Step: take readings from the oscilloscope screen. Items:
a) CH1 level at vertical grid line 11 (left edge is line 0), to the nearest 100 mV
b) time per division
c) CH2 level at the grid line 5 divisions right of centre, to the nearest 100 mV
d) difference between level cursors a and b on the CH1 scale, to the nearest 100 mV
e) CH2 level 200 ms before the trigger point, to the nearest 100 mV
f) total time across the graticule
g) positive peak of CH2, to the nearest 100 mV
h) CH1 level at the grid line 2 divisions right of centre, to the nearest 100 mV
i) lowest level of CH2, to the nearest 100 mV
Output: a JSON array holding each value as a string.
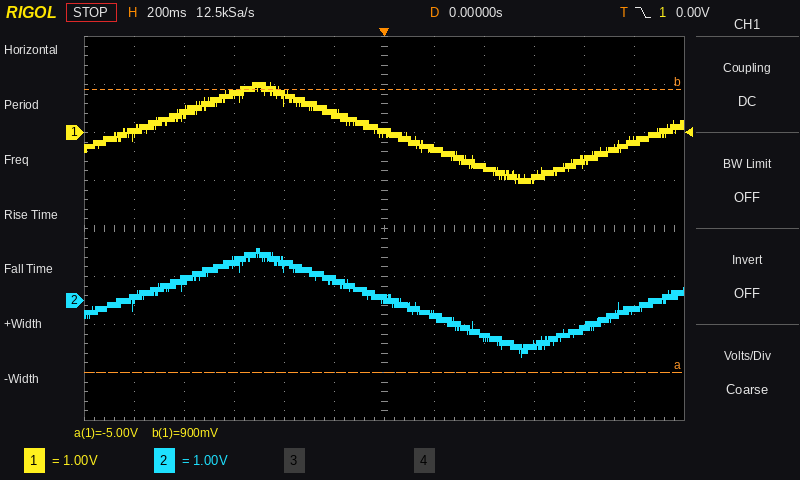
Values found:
["-200 mV", "200 ms", "-200 mV", "5.9 V", "400 mV", "2.4 s", "1.1 V", "-700 mV", "-1.2 V"]
